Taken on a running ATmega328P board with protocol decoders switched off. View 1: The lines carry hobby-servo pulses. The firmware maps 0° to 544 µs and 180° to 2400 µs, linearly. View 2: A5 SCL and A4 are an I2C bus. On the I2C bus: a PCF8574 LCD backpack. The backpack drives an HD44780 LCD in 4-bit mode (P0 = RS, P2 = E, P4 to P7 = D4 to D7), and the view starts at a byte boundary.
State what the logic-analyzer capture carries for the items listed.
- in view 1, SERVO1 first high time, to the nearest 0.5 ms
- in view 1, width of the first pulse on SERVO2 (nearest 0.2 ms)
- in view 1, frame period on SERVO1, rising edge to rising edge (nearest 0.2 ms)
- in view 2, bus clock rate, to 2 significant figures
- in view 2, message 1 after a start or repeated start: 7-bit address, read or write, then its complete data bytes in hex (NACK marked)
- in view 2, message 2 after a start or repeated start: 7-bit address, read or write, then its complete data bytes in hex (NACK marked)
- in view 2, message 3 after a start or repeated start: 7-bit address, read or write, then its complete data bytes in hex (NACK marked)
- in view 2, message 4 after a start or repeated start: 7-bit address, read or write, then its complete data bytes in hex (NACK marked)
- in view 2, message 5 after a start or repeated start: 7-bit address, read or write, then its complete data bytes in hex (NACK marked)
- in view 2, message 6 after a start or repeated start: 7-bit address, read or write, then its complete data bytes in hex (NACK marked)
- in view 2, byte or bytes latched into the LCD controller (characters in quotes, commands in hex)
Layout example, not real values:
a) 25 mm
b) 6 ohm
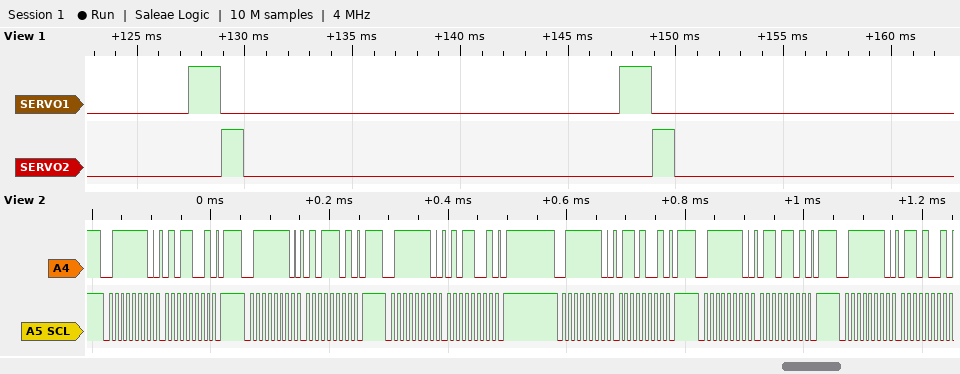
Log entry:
a) 1.5 ms
b) 1.0 ms
c) 20.0 ms
d) 100 kHz
e) 0x3F write: 59
f) 0x3F write: 5D
g) 0x3F write: 59
h) 0x3F write: 69
i) 0x3F write: 6D
j) 0x3F write: 69
k) 'V'
